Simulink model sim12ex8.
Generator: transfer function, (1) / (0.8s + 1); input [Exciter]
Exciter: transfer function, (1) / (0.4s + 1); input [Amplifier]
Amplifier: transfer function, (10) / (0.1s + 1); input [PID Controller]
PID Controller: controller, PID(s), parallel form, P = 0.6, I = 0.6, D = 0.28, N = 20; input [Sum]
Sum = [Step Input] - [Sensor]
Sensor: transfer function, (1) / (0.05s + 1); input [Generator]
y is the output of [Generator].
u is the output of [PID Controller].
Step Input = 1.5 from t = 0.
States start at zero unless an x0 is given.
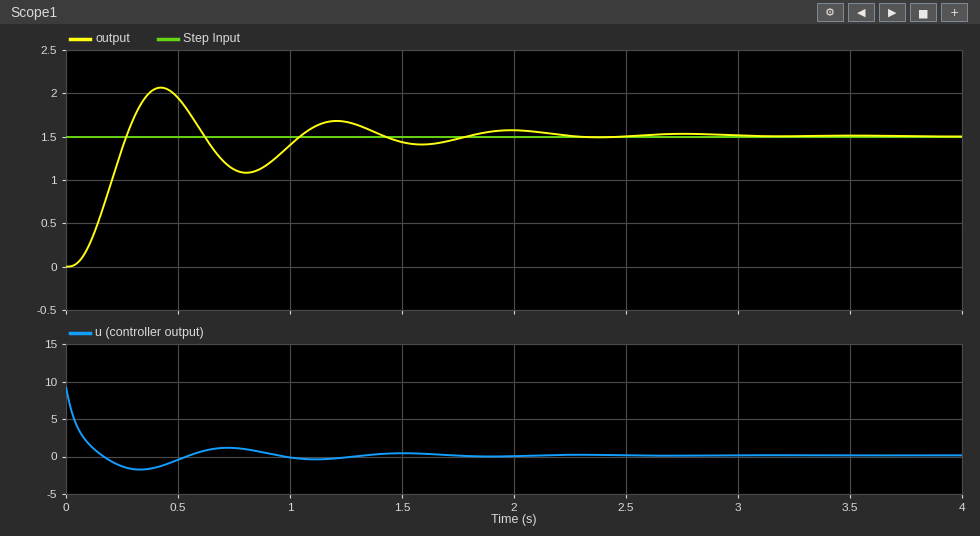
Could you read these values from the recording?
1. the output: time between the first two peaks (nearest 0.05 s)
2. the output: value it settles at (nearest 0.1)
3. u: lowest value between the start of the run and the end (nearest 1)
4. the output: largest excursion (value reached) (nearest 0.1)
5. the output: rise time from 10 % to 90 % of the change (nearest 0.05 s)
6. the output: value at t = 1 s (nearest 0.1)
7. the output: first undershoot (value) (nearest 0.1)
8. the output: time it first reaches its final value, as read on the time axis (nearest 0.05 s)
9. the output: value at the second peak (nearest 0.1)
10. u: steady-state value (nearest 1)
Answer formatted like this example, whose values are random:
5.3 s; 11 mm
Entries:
0.80 s; 1.5; -2; 2.1; 0.15 s; 1.4; 1.1; 0.25 s; 1.7; 0
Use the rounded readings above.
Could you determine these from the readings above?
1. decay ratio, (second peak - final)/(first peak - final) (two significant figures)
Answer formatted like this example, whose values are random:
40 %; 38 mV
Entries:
0.33
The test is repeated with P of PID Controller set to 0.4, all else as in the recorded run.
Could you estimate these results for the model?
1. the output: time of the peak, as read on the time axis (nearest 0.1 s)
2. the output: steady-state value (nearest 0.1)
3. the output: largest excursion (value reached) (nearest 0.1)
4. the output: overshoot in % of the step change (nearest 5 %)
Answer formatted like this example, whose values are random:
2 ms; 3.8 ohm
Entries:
0.4 s; 1.5; 1.9; 25 %
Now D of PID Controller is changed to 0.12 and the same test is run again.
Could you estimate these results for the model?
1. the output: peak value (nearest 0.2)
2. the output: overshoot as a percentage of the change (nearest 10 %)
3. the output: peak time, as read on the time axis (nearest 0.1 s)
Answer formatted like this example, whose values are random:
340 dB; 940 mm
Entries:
2.0; 40 %; 0.6 s
